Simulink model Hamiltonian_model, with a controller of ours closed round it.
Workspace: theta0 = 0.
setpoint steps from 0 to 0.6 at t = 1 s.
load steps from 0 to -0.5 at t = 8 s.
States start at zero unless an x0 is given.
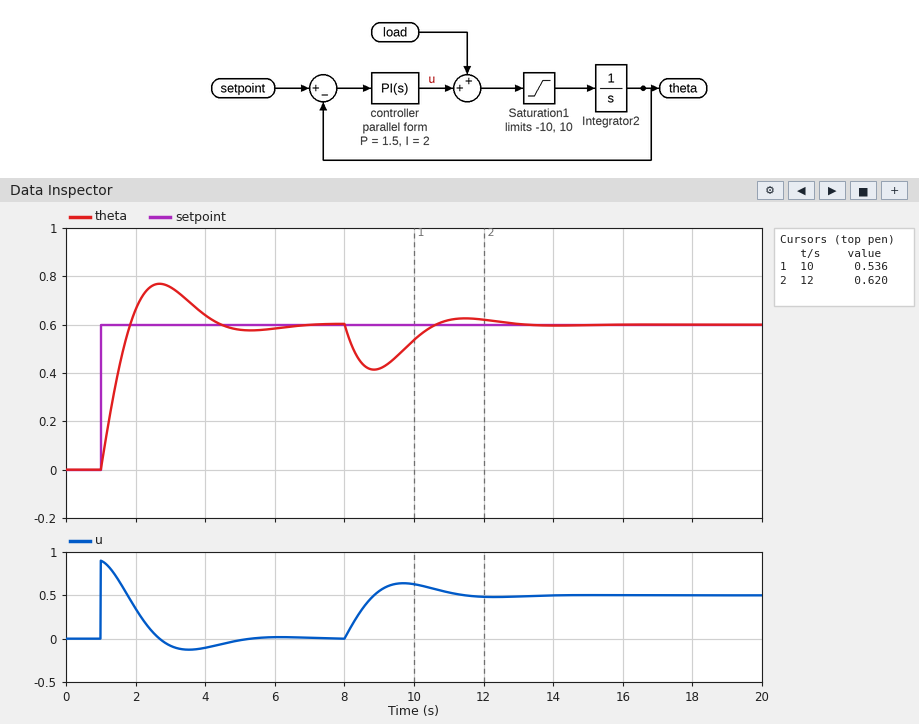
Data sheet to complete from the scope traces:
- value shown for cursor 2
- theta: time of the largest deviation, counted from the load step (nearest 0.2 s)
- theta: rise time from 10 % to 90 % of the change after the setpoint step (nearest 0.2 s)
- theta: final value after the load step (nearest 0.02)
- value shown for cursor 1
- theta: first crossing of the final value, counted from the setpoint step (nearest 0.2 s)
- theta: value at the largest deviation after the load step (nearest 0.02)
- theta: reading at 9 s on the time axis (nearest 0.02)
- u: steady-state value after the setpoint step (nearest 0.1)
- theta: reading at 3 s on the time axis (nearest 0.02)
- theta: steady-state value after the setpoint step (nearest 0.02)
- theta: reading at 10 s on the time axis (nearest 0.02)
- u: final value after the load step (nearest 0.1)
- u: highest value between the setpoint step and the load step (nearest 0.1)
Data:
0.620
0.8 s
0.6 s
0.60
0.536
0.8 s
0.42
0.42
0.0
0.76
0.60
0.54
0.5
0.9
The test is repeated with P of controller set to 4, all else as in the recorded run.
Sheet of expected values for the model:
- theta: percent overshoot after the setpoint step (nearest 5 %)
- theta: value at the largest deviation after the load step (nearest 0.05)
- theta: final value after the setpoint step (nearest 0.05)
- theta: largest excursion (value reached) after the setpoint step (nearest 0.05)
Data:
10 %
0.50
0.60
0.65
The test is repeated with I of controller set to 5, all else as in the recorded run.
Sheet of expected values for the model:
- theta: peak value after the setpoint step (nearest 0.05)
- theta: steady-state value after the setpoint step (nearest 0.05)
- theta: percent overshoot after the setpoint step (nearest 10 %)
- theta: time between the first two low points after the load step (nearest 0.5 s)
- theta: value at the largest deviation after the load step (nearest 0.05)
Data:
0.85
0.60
40 %
3.0 s
0.45
